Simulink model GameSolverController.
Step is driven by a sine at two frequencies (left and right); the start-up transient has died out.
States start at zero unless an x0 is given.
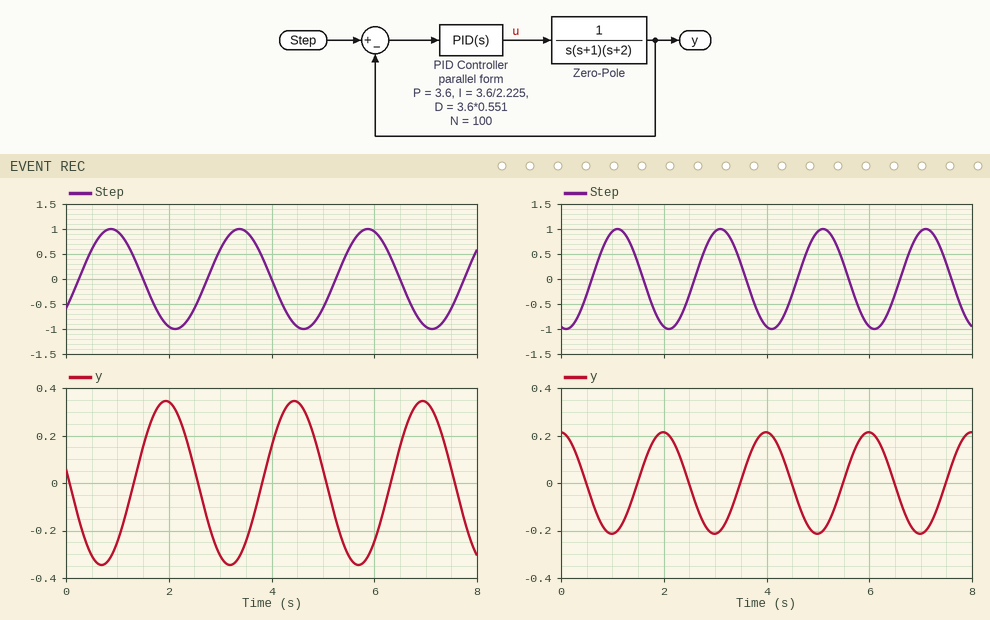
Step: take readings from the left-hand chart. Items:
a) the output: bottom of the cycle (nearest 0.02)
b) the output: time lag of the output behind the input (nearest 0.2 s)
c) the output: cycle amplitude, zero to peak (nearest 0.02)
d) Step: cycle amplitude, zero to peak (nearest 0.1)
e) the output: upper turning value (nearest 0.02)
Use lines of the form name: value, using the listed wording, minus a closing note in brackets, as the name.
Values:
the output: bottom of the cycle: -0.34
the output: time lag of the output behind the input: 1.0 s
the output: cycle amplitude, zero to peak: 0.34
Step: cycle amplitude, zero to peak: 1.0
the output: upper turning value: 0.34
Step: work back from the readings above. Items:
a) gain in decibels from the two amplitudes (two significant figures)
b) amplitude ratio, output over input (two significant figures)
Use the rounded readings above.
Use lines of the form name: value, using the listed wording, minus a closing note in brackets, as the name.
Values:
gain in decibels from the two amplitudes: -9.4 dB
amplitude ratio, output over input: 0.34
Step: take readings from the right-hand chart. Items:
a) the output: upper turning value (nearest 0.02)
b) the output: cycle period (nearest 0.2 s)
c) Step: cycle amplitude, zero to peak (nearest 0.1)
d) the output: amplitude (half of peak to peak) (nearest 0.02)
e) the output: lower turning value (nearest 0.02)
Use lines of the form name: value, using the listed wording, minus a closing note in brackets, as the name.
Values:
the output: upper turning value: 0.22
the output: cycle period: 2.0 s
Step: cycle amplitude, zero to peak: 1.0
the output: amplitude (half of peak to peak): 0.22
the output: lower turning value: -0.22
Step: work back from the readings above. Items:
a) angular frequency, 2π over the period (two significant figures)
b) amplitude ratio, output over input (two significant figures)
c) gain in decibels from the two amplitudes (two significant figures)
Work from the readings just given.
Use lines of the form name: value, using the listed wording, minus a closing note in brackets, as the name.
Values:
angular frequency, 2π over the period: 3.1 rad/s
amplitude ratio, output over input: 0.22
gain in decibels from the two amplitudes: -13 dB
